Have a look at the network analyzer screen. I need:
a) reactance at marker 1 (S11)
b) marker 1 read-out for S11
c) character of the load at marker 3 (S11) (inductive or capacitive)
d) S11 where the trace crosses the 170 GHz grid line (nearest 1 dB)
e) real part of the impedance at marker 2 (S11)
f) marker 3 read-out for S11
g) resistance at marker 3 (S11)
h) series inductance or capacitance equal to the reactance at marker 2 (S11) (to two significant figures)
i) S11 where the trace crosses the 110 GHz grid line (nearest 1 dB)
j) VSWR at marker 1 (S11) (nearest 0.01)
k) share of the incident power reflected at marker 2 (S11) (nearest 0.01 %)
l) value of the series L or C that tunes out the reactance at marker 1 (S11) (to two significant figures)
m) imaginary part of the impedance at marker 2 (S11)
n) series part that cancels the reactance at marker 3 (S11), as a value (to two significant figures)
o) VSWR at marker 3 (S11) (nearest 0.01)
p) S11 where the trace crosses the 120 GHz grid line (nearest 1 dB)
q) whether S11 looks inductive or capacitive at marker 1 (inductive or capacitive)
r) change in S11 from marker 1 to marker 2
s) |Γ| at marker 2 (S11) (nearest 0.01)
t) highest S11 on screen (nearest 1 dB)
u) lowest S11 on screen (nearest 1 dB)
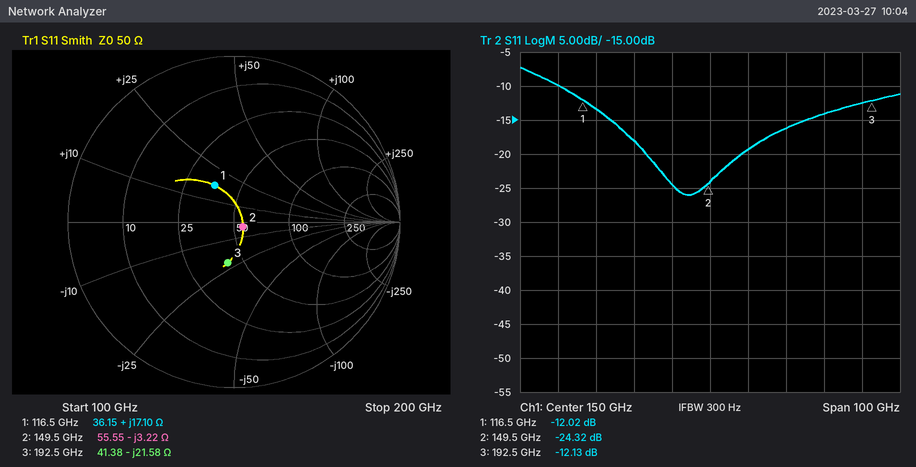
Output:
+17.10 Ω
-12.02 dB
capacitive
-16 dB
55.55 Ω
-12.13 dB
41.38 Ω
330 fF
-10 dB
1.67
0.37 %
80 fF
-3.22 Ω
18 pH
1.66
-13 dB
inductive
-12.30 dB
0.06
-7 dB
-26 dB
